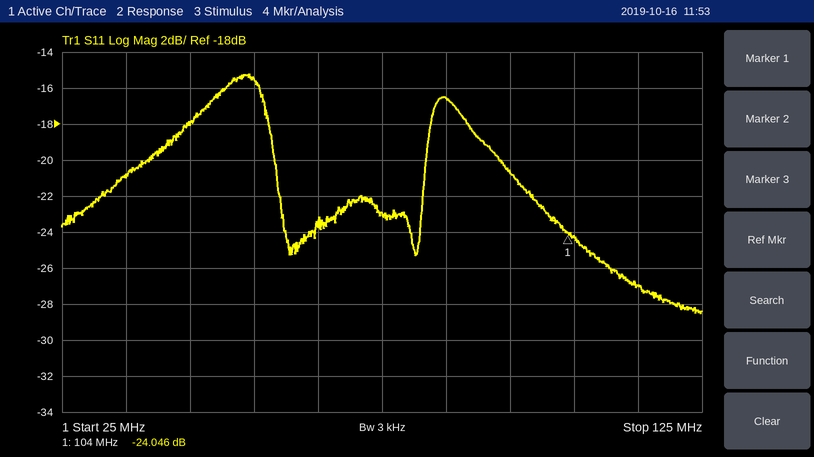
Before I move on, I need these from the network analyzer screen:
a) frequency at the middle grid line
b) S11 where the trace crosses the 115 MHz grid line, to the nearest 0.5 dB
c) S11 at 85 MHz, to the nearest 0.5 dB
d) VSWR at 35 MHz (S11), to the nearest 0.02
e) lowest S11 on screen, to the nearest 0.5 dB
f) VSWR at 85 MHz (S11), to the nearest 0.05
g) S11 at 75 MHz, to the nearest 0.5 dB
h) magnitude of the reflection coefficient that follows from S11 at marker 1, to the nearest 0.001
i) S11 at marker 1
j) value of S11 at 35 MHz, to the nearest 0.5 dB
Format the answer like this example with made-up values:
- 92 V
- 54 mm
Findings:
- 75 MHz
- -27.0 dB
- -16.5 dB
- 1.20
- -28.5 dB
- 1.35
- -23.0 dB
- 0.063
- -24.046 dB
- -21.0 dB
